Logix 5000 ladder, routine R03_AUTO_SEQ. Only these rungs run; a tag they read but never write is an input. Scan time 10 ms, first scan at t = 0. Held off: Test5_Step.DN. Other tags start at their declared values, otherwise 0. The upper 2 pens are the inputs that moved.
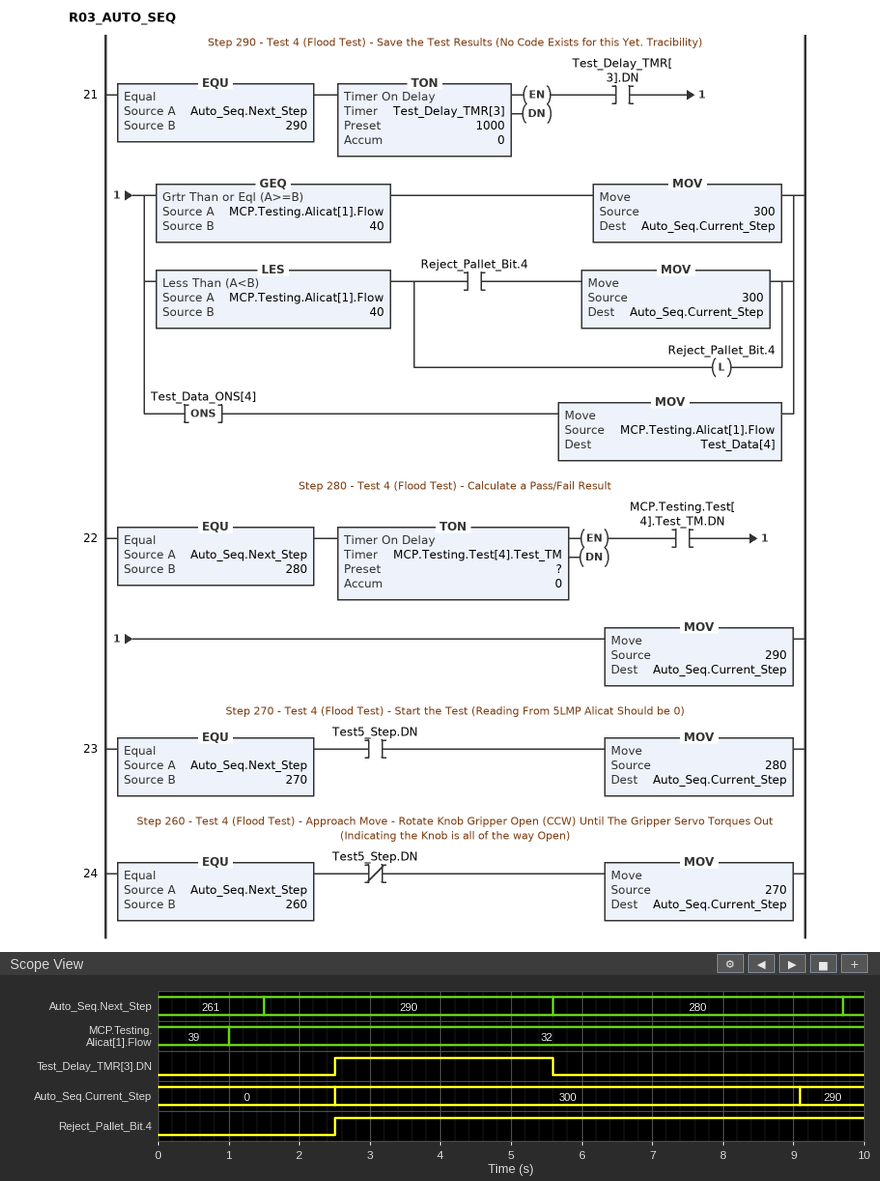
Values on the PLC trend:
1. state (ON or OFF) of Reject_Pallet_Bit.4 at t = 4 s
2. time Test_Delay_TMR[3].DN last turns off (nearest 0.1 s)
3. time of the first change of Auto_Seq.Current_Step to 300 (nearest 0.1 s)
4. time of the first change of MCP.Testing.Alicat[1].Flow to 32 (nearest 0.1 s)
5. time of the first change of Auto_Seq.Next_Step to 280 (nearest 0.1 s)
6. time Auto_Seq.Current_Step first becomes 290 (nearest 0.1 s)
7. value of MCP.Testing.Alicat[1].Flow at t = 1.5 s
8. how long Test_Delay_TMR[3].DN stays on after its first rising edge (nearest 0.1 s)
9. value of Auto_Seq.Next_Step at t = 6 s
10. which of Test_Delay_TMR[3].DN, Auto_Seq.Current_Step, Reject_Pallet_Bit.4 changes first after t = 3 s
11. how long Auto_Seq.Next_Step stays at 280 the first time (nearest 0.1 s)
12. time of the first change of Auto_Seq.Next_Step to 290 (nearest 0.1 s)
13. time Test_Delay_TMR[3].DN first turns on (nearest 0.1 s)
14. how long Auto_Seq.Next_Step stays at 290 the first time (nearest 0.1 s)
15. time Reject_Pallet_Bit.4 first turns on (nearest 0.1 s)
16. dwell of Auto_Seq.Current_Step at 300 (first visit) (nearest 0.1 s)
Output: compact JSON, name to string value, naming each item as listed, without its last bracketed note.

{"state (ON or OFF) of Reject_Pallet_Bit.4 at t = 4 s": "ON", "time Test_Delay_TMR[3].DN last turns off": "5.6 s", "time of the first change of Auto_Seq.Current_Step to 300": "2.5 s", "time of the first change of MCP.Testing.Alicat[1].Flow to 32": "1.0 s", "time of the first change of Auto_Seq.Next_Step to 280": "5.6 s", "time Auto_Seq.Current_Step first becomes 290": "9.1 s", "value of MCP.Testing.Alicat[1].Flow at t = 1.5 s": "32", "how long Test_Delay_TMR[3].DN stays on after its first rising edge": "3.1 s", "value of Auto_Seq.Next_Step at t = 6 s": "280", "which of Test_Delay_TMR[3].DN, Auto_Seq.Current_Step, Reject_Pallet_Bit.4 changes first after t = 3 s": "Test_Delay_TMR[3].DN", "how long Auto_Seq.Next_Step stays at 280 the first time": "4.1 s", "time of the first change of Auto_Seq.Next_Step to 290": "1.5 s", "time Test_Delay_TMR[3].DN first turns on": "2.5 s", "how long Auto_Seq.Next_Step stays at 290 the first time": "4.1 s", "time Reject_Pallet_Bit.4 first turns on": "2.5 s", "dwell of Auto_Seq.Current_Step at 300 (first visit)": "6.6 s"}
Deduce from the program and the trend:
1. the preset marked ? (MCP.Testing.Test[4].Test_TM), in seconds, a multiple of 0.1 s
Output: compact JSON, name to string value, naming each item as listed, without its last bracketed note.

{"the preset marked ? (MCP.Testing.Test[4].Test_TM), in seconds, a multiple of 0.1 s": "3.5 s"}
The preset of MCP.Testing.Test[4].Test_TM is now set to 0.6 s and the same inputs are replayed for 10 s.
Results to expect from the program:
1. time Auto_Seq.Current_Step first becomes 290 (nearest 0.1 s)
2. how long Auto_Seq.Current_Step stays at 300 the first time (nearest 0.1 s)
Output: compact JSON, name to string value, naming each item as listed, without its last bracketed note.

{"time Auto_Seq.Current_Step first becomes 290": "6.2 s", "how long Auto_Seq.Current_Step stays at 300 the first time": "3.7 s"}
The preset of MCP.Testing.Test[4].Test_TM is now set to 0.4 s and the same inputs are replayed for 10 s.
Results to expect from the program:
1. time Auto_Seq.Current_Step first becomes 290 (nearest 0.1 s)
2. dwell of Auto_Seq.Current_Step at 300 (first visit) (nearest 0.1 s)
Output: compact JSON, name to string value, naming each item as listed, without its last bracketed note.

{"time Auto_Seq.Current_Step first becomes 290": "6.0 s", "dwell of Auto_Seq.Current_Step at 300 (first visit)": "3.5 s"}
